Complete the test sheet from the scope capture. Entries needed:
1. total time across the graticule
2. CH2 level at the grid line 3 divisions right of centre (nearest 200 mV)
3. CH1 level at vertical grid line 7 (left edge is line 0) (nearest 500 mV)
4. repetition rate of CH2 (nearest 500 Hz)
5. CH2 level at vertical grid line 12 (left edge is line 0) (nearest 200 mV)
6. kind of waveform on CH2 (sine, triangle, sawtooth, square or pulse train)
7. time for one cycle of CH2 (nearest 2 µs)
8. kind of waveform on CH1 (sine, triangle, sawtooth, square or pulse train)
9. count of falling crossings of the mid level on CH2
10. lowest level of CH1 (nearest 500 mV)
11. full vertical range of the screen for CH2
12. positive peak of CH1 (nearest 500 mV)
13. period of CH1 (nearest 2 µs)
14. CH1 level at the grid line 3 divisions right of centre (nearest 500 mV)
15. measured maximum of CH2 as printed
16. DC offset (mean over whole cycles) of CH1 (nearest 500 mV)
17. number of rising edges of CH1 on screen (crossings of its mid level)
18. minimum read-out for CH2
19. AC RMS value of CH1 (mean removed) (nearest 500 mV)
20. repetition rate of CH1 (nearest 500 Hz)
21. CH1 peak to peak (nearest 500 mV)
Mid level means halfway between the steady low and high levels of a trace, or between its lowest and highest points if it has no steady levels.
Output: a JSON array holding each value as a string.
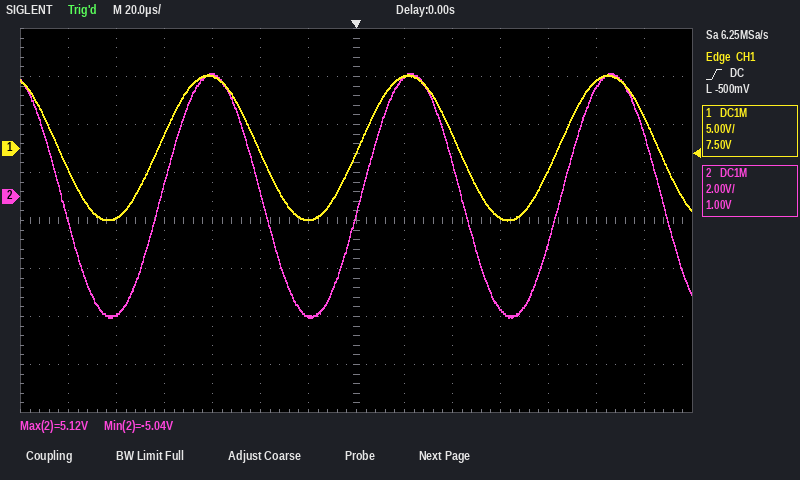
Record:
["280 µs", "-4.6 V", "-500 mV", "12.0 kHz", "4.6 V", "sine", "84 µs", "sine", "4", "-7.5 V", "16 V", "7.5 V", "84 µs", "-7.0 V", "5.12 V", "0.0 V", "3", "-5.04 V", "5.5 V", "12.0 kHz", "15.0 V"]
